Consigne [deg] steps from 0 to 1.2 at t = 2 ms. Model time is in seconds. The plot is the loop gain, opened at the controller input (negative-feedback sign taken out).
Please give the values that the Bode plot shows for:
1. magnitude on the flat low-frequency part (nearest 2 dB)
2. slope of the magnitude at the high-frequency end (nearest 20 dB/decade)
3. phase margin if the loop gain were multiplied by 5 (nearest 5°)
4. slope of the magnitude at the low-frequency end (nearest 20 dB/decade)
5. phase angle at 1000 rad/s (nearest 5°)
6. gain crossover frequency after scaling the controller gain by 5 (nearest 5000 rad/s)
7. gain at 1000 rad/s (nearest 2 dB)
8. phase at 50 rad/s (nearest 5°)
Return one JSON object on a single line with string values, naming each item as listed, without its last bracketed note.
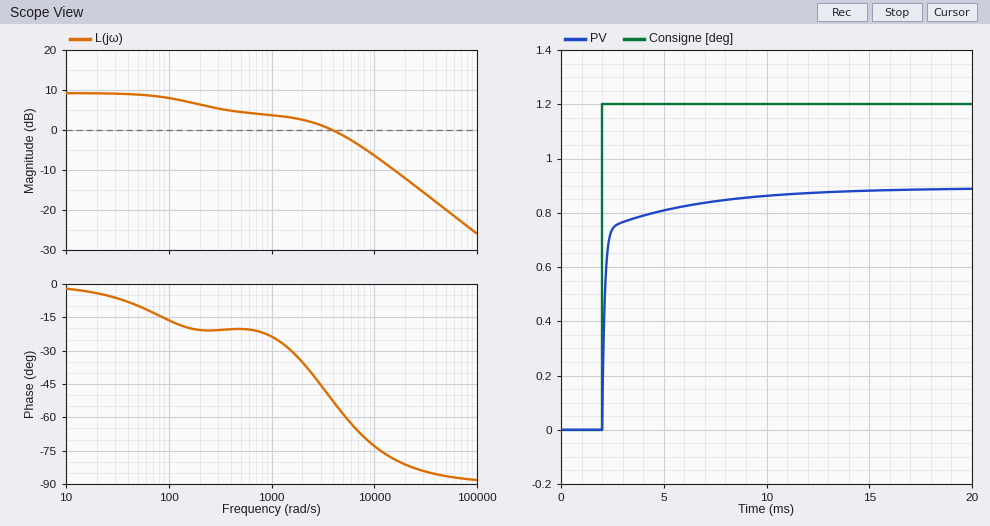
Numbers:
{"magnitude on the flat low-frequency part": "10 dB", "slope of the magnitude at the high-frequency end": "-20 dB/decade", "phase margin if the loop gain were multiplied by 5": "95°", "slope of the magnitude at the low-frequency end": "0 dB/decade", "phase angle at 1000 rad/s": "-25°", "gain crossover frequency after scaling the controller gain by 5": "25000 rad/s", "gain at 1000 rad/s": "4 dB", "phase at 50 rad/s": "-10°"}
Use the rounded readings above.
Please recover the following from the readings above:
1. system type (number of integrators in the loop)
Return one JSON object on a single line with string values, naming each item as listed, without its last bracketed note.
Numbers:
{"system type": "0"}
